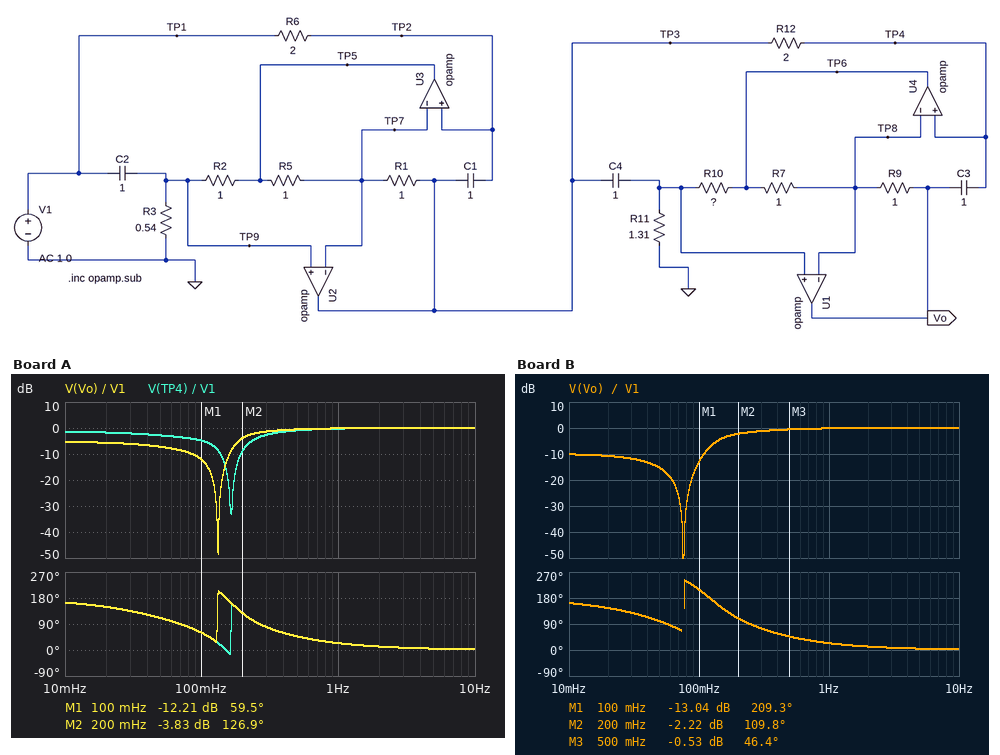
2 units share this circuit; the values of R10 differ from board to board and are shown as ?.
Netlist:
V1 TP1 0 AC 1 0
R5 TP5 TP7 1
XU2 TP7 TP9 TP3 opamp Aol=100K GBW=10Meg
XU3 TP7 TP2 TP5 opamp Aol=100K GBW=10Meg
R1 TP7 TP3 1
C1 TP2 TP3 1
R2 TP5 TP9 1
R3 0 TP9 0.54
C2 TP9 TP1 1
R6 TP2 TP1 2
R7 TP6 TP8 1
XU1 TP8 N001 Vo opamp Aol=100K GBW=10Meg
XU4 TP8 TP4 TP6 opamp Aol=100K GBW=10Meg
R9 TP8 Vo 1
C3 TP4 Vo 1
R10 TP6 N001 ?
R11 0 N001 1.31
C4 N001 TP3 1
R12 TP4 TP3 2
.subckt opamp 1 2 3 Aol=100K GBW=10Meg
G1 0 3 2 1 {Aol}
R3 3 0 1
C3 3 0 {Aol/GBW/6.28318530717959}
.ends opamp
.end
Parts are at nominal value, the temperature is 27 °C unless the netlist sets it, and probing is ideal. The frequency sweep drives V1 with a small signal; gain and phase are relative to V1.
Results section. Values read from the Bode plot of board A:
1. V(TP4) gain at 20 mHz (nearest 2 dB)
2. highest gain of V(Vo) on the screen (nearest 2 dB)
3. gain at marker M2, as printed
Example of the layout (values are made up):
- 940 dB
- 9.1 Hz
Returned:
- -2 dB
- 0 dB
- -3.83 dB
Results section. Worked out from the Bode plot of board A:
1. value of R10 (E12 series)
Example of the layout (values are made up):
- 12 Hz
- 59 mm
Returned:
- 0.47 Ω
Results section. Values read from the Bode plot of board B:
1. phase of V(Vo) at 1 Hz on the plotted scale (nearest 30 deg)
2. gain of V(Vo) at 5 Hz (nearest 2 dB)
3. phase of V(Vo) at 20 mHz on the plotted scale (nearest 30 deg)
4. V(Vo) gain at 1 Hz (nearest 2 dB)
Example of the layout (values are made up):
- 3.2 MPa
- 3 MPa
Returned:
- 30 deg
- 0 dB
- 150 deg
- 0 dB
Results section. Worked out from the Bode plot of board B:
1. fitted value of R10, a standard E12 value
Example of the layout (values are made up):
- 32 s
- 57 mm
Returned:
- 0.82 Ω
